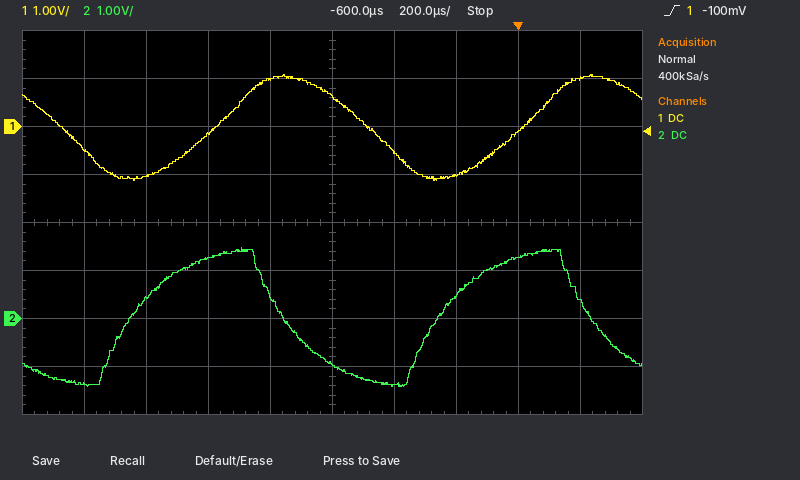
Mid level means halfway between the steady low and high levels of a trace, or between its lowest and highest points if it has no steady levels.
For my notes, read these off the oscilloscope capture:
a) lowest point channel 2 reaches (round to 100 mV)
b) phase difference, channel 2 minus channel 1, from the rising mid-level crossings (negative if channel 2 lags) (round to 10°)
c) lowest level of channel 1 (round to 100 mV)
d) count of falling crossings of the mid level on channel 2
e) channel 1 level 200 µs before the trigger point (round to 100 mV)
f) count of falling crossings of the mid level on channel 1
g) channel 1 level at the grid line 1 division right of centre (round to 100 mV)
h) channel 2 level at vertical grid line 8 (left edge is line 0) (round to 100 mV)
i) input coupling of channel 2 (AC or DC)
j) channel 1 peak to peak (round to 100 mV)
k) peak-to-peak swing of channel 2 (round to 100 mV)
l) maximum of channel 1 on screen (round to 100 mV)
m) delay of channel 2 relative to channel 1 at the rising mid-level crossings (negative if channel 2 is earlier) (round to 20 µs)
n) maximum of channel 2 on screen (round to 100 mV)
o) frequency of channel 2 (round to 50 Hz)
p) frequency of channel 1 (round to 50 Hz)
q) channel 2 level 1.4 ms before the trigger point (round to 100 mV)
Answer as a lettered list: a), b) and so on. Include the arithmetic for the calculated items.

a) -1.4 V
b) +100°
c) -1.1 V
d) 2
e) -1.0 V
f) 2
g) -500 mV
h) 1.3 V
i) DC
j) 1.1 V − (-1.1 V) = 2.2 V
k) 1.5 V − (-1.4 V) = 2.9 V
l) 1.1 V
m) -280 µs
n) 1.5 V
o) 1.00 kHz
p) 1.00 kHz
q) -1.4 V
